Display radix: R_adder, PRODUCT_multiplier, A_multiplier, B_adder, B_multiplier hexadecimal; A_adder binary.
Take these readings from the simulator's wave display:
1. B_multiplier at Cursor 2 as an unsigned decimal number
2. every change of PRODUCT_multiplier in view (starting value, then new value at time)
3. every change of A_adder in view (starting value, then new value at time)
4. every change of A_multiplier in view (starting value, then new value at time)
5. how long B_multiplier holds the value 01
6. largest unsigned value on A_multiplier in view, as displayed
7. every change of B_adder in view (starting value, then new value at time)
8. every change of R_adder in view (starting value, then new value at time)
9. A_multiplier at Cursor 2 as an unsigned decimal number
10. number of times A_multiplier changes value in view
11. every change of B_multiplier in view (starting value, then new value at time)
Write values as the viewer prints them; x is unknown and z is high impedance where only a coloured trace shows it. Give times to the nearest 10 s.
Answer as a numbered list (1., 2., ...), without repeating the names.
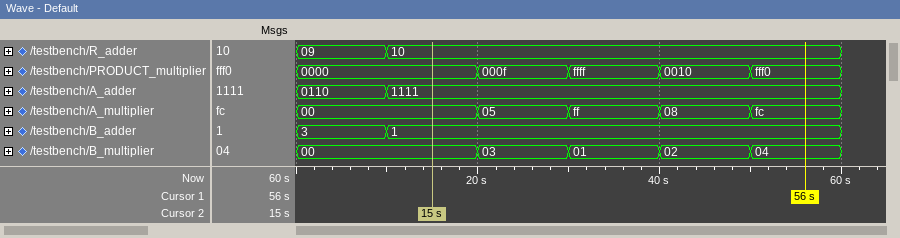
1. 0
2. 0000, 000f at 20 s, ffff at 30 s, 0010 at 40 s, fff0 at 50 s
3. 0110, 1111 at 10 s
4. 00, 05 at 20 s, ff at 30 s, 08 at 40 s, fc at 50 s
5. 10 s
6. ff
7. 3, 1 at 10 s
8. 09, 10 at 10 s
9. 0
10. 4
11. 00, 03 at 20 s, 01 at 30 s, 02 at 40 s, 04 at 50 s
